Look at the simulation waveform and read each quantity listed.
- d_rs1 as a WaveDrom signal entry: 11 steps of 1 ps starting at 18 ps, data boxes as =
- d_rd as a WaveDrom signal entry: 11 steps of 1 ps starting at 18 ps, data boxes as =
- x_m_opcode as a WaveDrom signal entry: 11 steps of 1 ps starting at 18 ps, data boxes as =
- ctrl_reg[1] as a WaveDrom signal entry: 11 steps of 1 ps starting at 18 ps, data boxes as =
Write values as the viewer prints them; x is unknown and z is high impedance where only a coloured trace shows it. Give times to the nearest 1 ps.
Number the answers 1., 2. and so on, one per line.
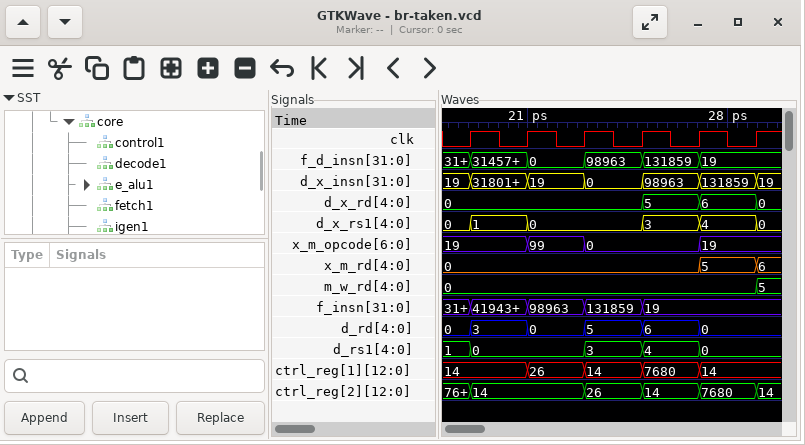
1. {name: 'd_rs1', wave: '==...=.=.=.', data: '1 0 3 4 0'}
2. {name: 'd_rd', wave: '==.=.=.=.=.', data: '0 3 0 5 6 0'}
3. {name: 'x_m_opcode', wave: '=..=.=...=.', data: '19 99 0 19'}
4. {name: 'ctrl_reg[1]', wave: '=..=.=.=.=.', data: '14 26 14 7680 14'}
